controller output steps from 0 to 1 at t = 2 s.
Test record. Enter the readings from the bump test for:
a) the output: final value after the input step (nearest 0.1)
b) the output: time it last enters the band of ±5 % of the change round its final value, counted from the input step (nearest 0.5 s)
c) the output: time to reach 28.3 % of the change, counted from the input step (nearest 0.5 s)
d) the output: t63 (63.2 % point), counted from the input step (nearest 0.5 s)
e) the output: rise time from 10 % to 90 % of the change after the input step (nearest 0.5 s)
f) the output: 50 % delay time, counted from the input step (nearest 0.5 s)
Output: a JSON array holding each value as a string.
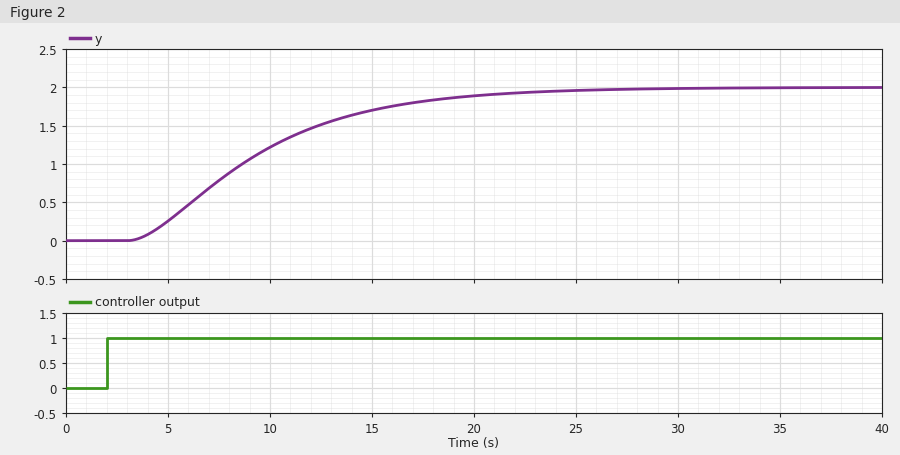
["2.0", "18.5 s", "4.5 s", "8.5 s", "12.5 s", "6.5 s"]
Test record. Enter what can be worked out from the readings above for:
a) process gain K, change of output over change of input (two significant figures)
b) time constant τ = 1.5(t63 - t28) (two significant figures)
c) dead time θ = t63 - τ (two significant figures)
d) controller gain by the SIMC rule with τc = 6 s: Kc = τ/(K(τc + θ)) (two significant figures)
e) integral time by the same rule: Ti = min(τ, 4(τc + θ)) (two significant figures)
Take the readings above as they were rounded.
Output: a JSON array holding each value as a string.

["2.0", "6.0 s", "2.5 s", "0.35", "6.0 s"]
